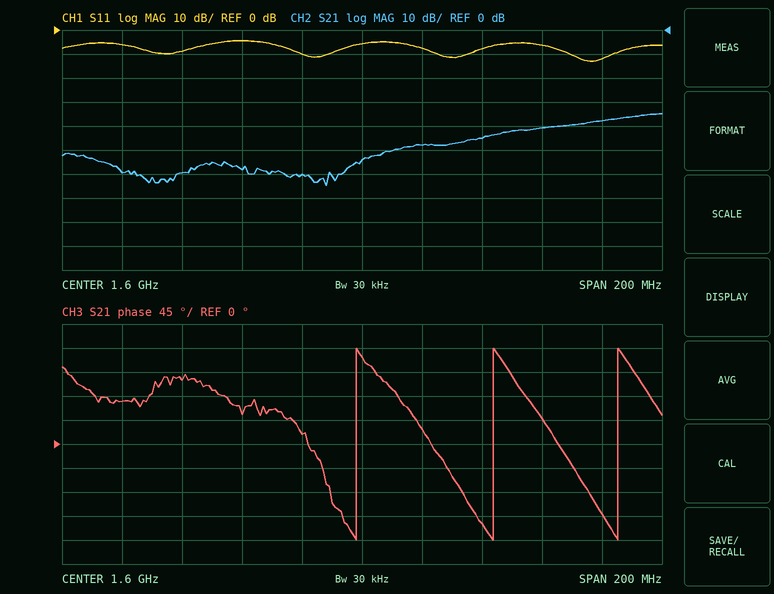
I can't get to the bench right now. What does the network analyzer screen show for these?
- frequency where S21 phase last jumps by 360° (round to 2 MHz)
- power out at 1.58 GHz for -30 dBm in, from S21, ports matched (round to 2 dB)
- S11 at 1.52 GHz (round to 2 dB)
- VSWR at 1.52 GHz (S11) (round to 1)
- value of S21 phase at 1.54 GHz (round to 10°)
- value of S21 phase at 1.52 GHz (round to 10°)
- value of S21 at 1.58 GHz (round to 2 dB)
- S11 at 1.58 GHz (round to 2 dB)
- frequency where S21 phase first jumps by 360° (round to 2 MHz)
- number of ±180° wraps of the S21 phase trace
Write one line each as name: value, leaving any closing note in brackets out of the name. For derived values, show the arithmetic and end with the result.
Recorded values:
frequency where S21 phase last jumps by 360°: 1.686 GHz
power out at 1.58 GHz for -30 dBm in, from S21, ports matched: -30 dBm + (-60 dB) = -90 dBm
S11 at 1.52 GHz: -6 dB
VSWR at 1.52 GHz (S11): |Γ| = 10^(-6/20) = 0.5012; VSWR = (1 + 0.5012)/(1 − 0.5012) ≈ 3
value of S21 phase at 1.54 GHz: 120°
value of S21 phase at 1.52 GHz: 80°
value of S21 at 1.58 GHz: -60 dB
S11 at 1.58 GHz: -10 dB
frequency where S21 phase first jumps by 360°: 1.598 GHz
number of ±180° wraps of the S21 phase trace: 3
